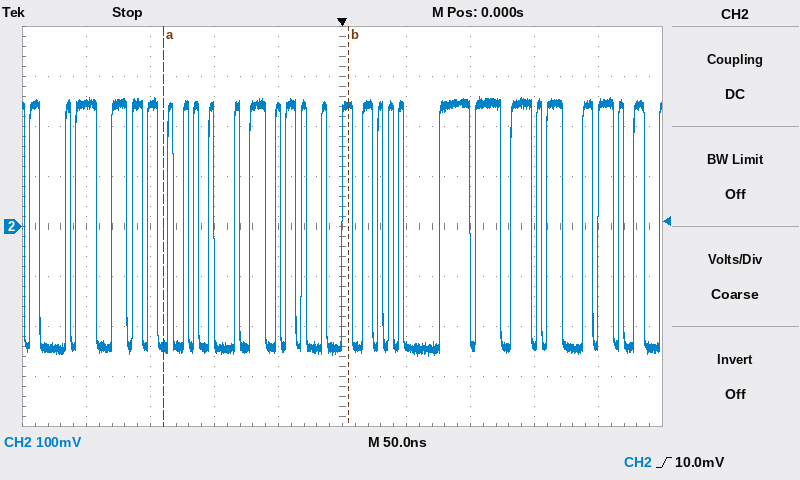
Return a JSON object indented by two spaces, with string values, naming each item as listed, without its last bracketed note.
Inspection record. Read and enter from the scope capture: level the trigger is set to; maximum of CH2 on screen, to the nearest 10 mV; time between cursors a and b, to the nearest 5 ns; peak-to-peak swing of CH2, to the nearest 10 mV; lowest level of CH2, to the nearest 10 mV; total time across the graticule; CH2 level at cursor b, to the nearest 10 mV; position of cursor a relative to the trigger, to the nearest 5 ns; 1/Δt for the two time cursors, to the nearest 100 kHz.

{
  "level the trigger is set to": "10.0 mV",
  "maximum of CH2 on screen, to the nearest 10 mV": "260 mV",
  "time between cursors a and b, to the nearest 5 ns": "145 ns",
  "peak-to-peak swing of CH2, to the nearest 10 mV": "520 mV",
  "lowest level of CH2, to the nearest 10 mV": "-260 mV",
  "total time across the graticule": "500 ns",
  "CH2 level at cursor b, to the nearest 10 mV": "240 mV",
  "position of cursor a relative to the trigger, to the nearest 5 ns": "-140 ns",
  "1/Δt for the two time cursors, to the nearest 100 kHz": "6.9 MHz"
}
